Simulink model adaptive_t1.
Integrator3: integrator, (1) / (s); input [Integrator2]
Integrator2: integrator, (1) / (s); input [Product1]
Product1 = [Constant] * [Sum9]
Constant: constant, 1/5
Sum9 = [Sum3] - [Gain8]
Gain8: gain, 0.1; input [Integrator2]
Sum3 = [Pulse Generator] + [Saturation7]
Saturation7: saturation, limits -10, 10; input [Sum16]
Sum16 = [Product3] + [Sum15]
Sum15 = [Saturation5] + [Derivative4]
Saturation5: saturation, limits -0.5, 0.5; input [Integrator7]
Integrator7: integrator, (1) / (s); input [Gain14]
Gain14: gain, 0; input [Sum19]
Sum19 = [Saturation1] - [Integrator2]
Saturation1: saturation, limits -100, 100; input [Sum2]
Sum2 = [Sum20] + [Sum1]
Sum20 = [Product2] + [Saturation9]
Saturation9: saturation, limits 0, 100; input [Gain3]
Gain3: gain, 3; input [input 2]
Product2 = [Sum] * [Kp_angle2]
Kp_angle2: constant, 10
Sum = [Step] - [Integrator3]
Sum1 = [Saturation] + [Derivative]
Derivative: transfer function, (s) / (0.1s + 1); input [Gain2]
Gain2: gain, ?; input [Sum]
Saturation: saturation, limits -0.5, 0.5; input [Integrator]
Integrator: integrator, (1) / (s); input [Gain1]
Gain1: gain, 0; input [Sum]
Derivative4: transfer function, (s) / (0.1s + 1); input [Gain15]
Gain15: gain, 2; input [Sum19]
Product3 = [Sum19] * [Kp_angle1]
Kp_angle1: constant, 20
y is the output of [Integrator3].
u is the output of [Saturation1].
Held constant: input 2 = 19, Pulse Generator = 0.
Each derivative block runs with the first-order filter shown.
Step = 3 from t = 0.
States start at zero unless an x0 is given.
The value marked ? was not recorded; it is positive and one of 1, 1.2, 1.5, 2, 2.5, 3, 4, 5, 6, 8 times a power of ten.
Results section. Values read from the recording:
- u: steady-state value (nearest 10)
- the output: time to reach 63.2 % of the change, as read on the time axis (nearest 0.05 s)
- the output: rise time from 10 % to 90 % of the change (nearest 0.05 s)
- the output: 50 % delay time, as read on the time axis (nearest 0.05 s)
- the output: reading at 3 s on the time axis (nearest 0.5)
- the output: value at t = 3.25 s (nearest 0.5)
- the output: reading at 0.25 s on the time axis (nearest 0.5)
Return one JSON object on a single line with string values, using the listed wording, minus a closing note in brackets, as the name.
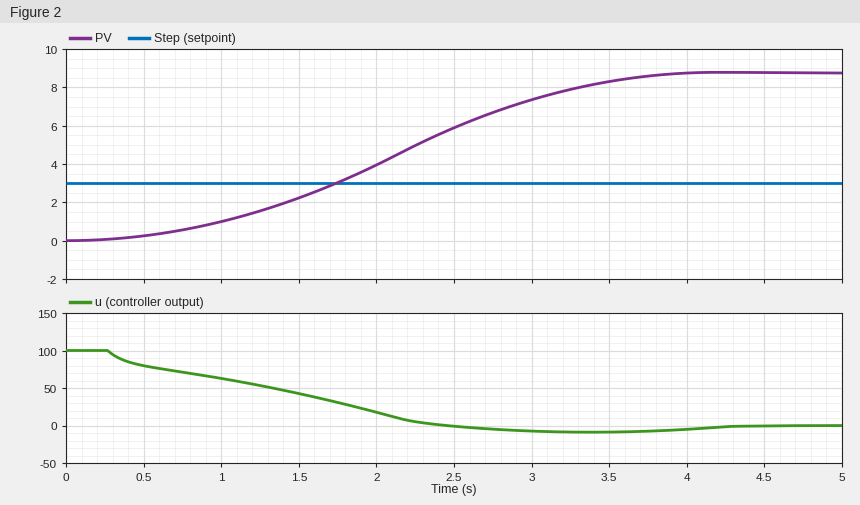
{"u: steady-state value": "0", "the output: time to reach 63.2 % of the change, as read on the time axis": "2.40 s", "the output: rise time from 10 % to 90 % of the change": "2.30 s", "the output: 50 % delay time, as read on the time axis": "2.10 s", "the output: reading at 3 s on the time axis": "7.5", "the output: value at t = 3.25 s": "8.0", "the output: reading at 0.25 s on the time axis": "0.0"}
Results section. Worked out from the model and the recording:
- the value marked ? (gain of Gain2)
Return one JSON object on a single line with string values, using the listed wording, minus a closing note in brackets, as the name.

{"the value marked ?": "8"}
